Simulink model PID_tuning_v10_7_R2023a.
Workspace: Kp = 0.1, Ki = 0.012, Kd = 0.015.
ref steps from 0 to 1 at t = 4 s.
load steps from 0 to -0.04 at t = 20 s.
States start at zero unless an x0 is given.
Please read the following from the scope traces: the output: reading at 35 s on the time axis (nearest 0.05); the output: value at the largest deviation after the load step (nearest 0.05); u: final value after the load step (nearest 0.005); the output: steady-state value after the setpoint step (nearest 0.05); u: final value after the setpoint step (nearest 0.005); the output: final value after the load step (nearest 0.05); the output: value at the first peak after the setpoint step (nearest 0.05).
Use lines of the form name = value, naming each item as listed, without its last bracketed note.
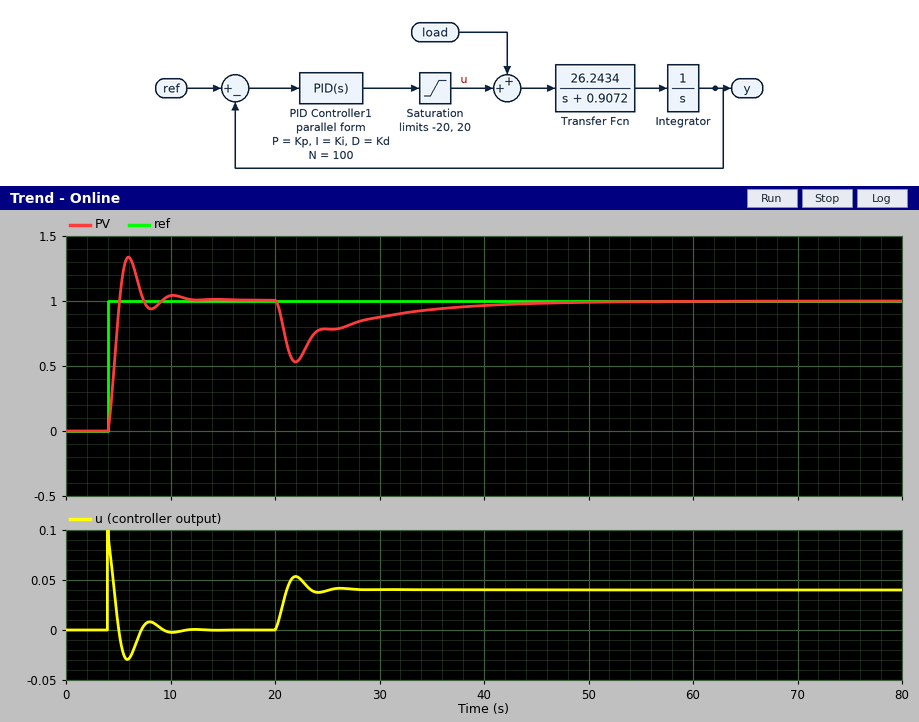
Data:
the output: reading at 35 s on the time axis = 0.95
the output: value at the largest deviation after the load step = 0.55
u: final value after the load step = 0.040
the output: steady-state value after the setpoint step = 1.00
u: final value after the setpoint step = 0.000
the output: final value after the load step = 1.00
the output: value at the first peak after the setpoint step = 1.35
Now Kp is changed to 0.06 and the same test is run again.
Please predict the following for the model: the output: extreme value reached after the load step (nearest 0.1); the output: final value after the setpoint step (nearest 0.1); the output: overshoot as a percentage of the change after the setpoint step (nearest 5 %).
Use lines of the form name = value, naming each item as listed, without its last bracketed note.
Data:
the output: extreme value reached after the load step = 0.3
the output: final value after the setpoint step = 1.0
the output: overshoot as a percentage of the change after the setpoint step = 30 %
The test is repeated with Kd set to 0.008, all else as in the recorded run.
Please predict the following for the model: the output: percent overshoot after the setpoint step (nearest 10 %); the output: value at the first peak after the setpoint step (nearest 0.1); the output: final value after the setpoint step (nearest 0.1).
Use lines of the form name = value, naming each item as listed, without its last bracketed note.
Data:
the output: percent overshoot after the setpoint step = 40 %
the output: value at the first peak after the setpoint step = 1.4
the output: final value after the setpoint step = 1.0
